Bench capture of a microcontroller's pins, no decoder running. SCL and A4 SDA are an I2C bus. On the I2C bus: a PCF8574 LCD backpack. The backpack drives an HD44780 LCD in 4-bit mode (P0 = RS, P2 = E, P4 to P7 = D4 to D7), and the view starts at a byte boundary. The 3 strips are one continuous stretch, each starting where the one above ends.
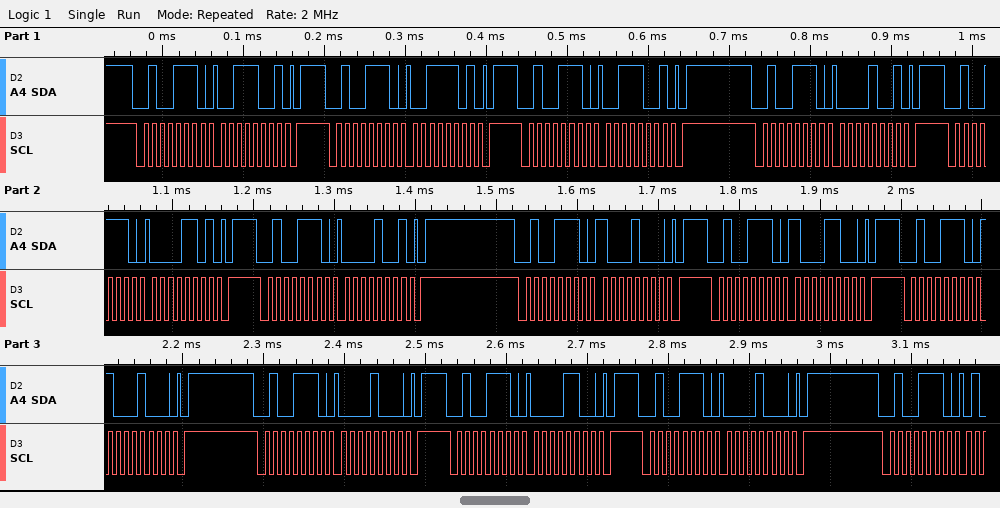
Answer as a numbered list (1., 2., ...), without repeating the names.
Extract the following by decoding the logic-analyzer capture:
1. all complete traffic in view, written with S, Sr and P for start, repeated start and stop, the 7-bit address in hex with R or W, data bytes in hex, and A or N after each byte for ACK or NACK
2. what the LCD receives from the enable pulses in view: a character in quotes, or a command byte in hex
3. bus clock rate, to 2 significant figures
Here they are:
1. S 27W A 39 A P S 27W A 3D A P S 27W A 39 A P S 27W A 09 A P S 27W A 0D A P S 27W A 09 A P S 27W A 88 A P S 27W A 8C A P S 27W A 88 A P S 27W A 08 A P S 27W A 0C A P S 27W A 08 A P S 27W A
2. '0' 0x80
3. 100 kHz
